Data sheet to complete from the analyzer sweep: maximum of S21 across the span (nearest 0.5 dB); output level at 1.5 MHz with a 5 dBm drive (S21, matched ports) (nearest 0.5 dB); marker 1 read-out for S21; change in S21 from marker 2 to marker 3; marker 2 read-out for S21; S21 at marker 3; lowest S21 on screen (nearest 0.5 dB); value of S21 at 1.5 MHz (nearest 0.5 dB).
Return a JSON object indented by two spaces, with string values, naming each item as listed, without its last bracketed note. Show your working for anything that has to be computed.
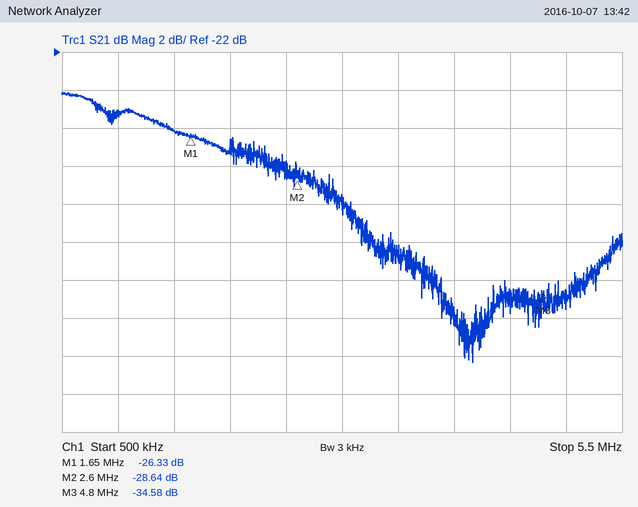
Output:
{
  "maximum of S21 across the span": "-24.0 dB",
  "output level at 1.5 MHz with a 5 dBm drive (S21, matched ports)": "5 dBm + (-26.0 dB) = -21.0 dBm",
  "marker 1 read-out for S21": "-26.33 dB",
  "change in S21 from marker 2 to marker 3": "-34.58 − (-28.64) = -5.94 dB",
  "marker 2 read-out for S21": "-28.64 dB",
  "S21 at marker 3": "-34.58 dB",
  "lowest S21 on screen": "-38.5 dB",
  "value of S21 at 1.5 MHz": "-26.0 dB"
}
